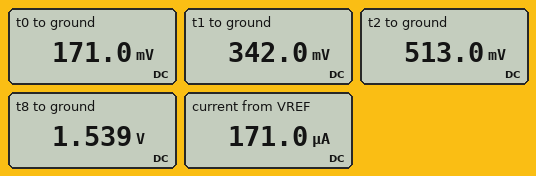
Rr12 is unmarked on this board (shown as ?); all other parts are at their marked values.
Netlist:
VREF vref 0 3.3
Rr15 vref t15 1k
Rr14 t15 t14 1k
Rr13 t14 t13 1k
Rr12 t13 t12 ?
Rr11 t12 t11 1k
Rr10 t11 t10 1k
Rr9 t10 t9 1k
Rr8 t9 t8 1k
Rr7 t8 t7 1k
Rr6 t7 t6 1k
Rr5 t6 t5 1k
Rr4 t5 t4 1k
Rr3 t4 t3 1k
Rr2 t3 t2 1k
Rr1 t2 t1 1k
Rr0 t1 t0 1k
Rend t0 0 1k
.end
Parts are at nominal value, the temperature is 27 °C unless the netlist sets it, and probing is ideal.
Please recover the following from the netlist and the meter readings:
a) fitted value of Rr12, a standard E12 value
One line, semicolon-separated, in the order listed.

3.3 kΩ
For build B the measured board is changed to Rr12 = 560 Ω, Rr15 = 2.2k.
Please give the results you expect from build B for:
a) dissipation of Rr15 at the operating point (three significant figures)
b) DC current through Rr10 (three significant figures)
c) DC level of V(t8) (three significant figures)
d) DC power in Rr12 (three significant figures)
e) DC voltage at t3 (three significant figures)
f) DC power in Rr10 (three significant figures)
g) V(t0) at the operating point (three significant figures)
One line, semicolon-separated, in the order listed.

76.0 µW; 186 µA; 1.67 V; 19.3 µW; 743 mV; 34.5 µW; 186 mV
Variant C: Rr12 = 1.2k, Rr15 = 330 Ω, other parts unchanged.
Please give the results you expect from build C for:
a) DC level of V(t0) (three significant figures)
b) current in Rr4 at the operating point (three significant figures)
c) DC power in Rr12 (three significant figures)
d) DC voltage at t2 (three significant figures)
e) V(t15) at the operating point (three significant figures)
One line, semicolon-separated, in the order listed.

200 mV; 200 µA; 47.8 µW; 599 mV; 3.23 V
